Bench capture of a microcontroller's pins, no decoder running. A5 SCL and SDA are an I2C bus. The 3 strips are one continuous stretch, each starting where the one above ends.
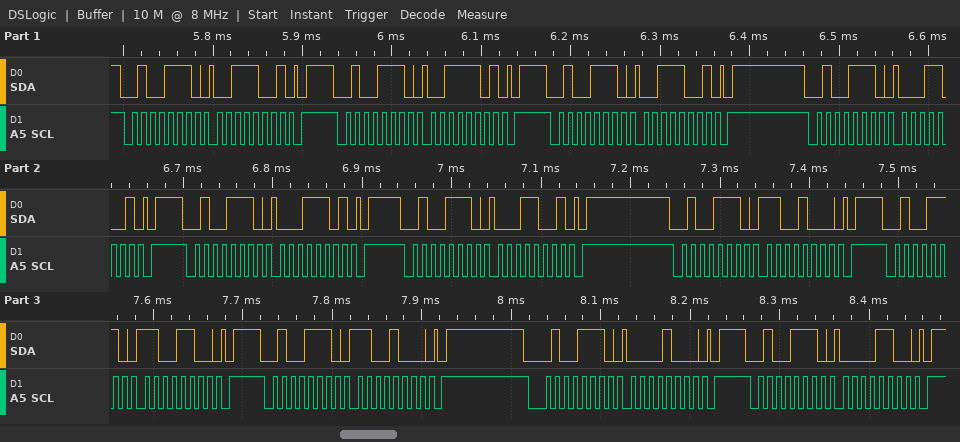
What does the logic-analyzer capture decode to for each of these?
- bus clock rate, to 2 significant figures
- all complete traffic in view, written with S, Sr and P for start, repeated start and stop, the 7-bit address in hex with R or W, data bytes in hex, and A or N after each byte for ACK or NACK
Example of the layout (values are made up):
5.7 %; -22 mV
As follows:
100 kHz; S 27W A 39 A P S 27W A 3D A P S 27W A 39 A P S 27W A 19 A P S 27W A 1D A P S 27W A 19 A P S 27W A C8 A P S 27W A CC A P S 27W A C8 A P S 27W A 08 A P S 27W A 0C A P
